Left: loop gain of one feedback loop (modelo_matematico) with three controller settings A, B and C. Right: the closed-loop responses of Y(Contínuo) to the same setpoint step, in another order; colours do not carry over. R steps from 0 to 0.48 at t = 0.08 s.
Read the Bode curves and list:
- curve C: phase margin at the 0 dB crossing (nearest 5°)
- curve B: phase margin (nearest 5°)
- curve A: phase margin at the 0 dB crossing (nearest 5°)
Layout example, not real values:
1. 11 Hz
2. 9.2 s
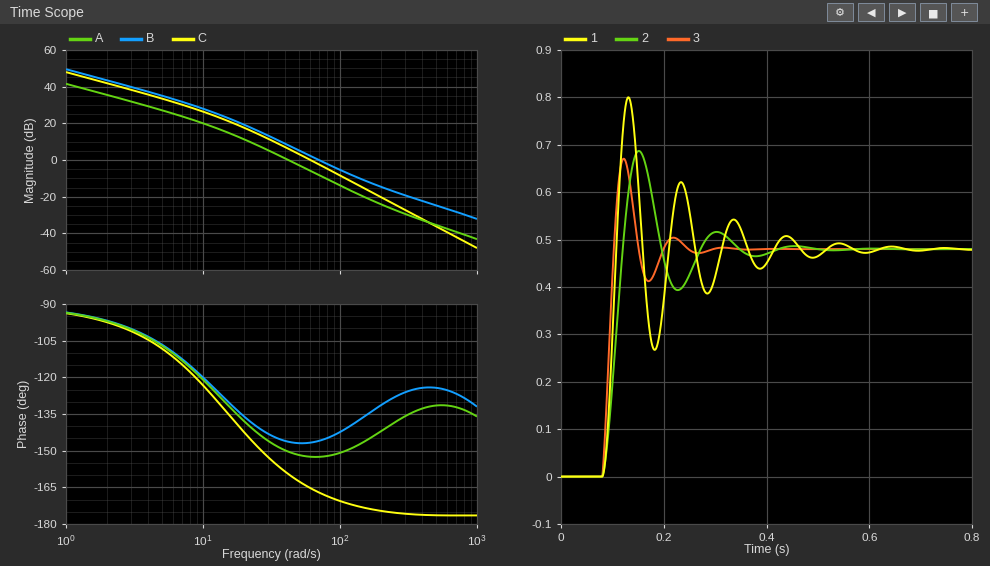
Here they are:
1. 15°
2. 35°
3. 30°
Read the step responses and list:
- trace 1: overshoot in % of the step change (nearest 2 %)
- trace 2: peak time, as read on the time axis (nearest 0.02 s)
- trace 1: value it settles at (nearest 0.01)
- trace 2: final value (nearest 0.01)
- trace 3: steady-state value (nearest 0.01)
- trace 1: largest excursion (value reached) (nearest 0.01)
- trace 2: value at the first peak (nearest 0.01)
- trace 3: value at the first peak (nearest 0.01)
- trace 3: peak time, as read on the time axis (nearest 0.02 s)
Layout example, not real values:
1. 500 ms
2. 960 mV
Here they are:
1. 66 %
2. 0.16 s
3. 0.48
4. 0.48
5. 0.48
6. 0.80
7. 0.69
8. 0.67
9. 0.12 s
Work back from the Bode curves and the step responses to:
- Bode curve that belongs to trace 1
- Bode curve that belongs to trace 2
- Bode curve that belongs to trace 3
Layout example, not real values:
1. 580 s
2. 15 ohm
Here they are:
1. C
2. A
3. B
